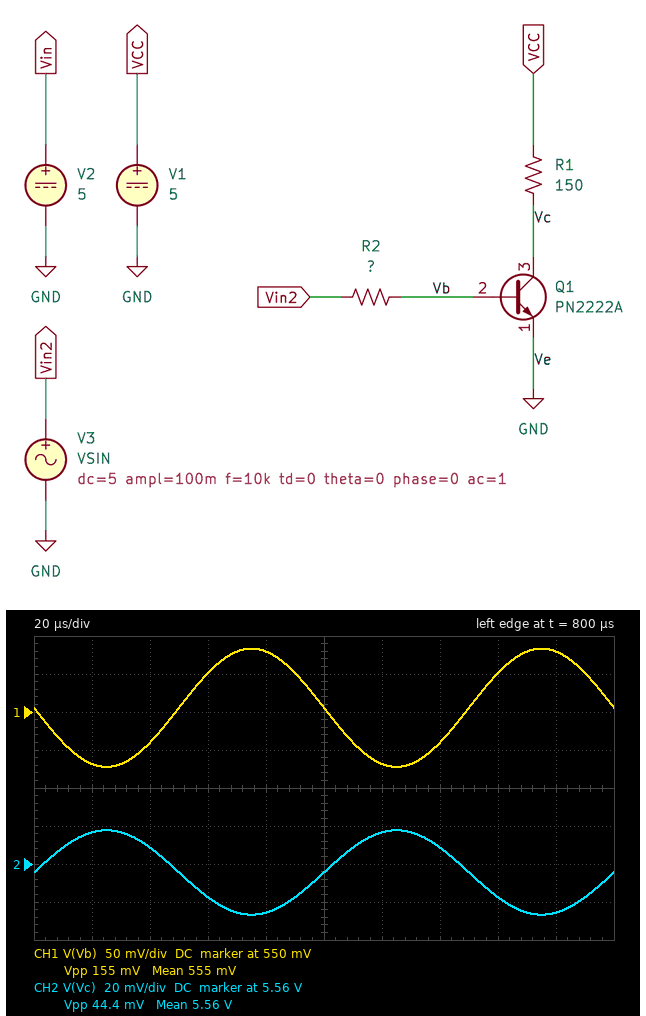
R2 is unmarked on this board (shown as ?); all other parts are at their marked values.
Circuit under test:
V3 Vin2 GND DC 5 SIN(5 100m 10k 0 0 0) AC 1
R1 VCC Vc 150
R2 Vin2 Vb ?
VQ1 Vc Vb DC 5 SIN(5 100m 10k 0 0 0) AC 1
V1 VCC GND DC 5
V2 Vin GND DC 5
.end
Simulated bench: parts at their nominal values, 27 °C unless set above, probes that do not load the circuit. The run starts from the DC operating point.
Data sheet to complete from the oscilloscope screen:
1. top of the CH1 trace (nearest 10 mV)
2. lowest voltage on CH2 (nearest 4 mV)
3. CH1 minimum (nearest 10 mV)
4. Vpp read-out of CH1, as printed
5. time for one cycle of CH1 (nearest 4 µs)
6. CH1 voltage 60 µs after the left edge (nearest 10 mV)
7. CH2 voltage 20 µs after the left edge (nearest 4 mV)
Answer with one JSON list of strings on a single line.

["630 mV", "5.532 V", "480 mV", "155 mV", "100 µs", "600 mV", "5.576 V"]
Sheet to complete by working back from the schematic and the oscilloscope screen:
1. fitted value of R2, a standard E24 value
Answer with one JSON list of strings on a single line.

["1.2 kΩ"]
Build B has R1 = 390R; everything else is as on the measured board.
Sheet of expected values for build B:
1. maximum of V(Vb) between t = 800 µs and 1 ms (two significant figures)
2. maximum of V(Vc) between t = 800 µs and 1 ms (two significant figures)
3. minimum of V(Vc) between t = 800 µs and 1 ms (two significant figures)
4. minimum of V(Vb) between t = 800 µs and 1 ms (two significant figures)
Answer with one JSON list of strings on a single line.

["1.3 V", "6.3 V", "6.2 V", "1.2 V"]
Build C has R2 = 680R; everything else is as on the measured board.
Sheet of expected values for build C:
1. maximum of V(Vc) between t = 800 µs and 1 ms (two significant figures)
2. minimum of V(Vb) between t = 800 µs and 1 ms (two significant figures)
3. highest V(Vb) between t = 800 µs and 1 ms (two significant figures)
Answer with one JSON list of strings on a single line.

["5.9 V", "840 mV", "970 mV"]
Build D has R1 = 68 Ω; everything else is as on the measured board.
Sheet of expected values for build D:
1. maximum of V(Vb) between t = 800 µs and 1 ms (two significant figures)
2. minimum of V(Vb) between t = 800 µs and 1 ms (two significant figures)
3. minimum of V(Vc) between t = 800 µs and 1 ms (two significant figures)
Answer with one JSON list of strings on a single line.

["360 mV", "180 mV", "5.3 V"]
